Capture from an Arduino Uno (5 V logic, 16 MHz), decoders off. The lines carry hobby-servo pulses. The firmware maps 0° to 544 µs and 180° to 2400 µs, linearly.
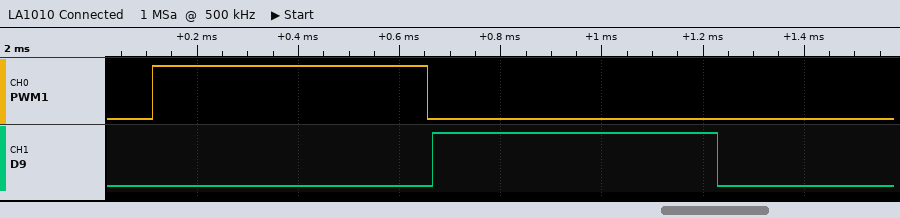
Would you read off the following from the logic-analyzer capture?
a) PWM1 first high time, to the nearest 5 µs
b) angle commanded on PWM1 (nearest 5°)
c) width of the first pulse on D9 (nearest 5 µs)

545 µs
0°
565 µs
